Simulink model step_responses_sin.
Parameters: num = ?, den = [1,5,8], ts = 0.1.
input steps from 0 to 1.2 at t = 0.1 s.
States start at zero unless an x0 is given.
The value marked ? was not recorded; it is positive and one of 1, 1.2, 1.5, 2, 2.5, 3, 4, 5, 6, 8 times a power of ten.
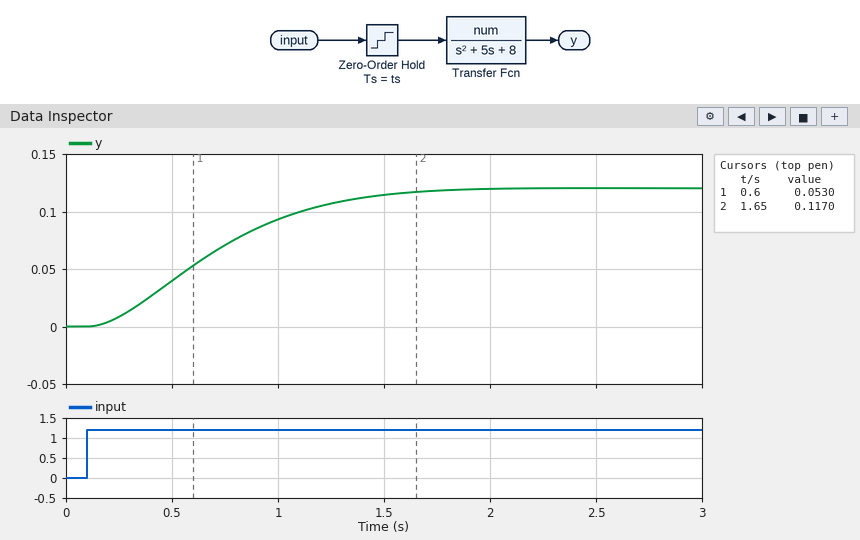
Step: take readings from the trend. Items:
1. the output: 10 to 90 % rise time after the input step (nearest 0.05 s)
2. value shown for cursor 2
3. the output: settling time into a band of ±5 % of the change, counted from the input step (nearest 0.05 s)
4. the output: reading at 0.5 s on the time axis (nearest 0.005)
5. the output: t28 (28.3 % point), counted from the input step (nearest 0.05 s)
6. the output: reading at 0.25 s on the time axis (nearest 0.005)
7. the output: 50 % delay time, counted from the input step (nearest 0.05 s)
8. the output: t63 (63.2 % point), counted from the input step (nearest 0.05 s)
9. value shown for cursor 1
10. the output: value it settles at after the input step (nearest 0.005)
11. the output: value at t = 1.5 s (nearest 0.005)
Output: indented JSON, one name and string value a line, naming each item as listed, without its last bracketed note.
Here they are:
{
  "the output: 10 to 90 % rise time after the input step": "1.00 s",
  "value shown for cursor 2": "0.1170",
  "the output: settling time into a band of ±5 % of the change, counted from the input step": "1.40 s",
  "the output: reading at 0.5 s on the time axis": "0.040",
  "the output: t28 (28.3 % point), counted from the input step": "0.35 s",
  "the output: reading at 0.25 s on the time axis": "0.010",
  "the output: 50 % delay time, counted from the input step": "0.55 s",
  "the output: t63 (63.2 % point), counted from the input step": "0.70 s",
  "value shown for cursor 1": "0.0530",
  "the output: value it settles at after the input step": "0.120",
  "the output: value at t = 1.5 s": "0.115"
}
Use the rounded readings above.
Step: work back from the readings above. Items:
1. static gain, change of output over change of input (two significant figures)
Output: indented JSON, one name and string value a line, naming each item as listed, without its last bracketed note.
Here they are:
{
  "static gain, change of output over change of input": "0.10"
}
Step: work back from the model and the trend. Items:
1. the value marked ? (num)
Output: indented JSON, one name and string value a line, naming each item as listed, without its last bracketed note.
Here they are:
{
  "the value marked ?": "0.8"
}
